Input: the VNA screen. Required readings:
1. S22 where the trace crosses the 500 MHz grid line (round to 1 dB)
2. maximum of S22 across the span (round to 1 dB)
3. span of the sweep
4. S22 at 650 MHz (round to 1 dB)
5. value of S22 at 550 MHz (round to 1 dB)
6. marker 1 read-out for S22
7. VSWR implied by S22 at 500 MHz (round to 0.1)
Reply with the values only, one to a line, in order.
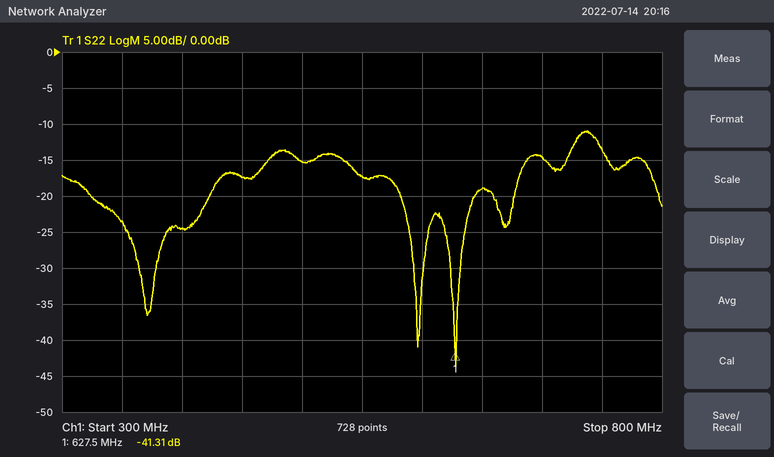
-15 dB
-11 dB
500 MHz
-19 dB
-17 dB
-41.31 dB
1.4
